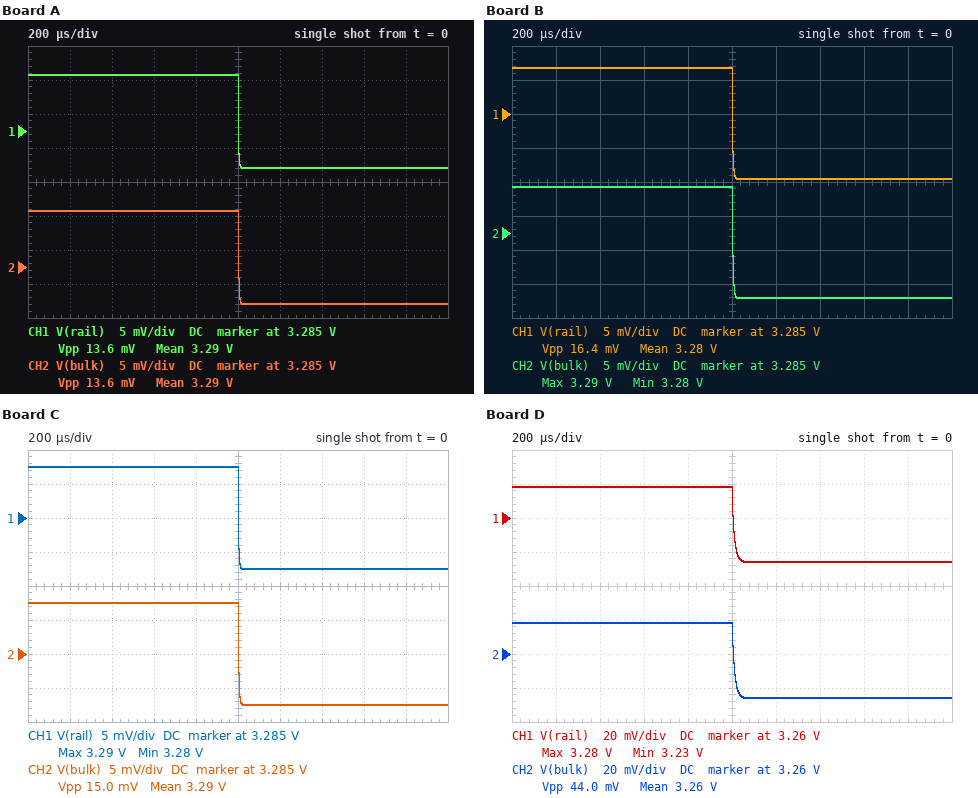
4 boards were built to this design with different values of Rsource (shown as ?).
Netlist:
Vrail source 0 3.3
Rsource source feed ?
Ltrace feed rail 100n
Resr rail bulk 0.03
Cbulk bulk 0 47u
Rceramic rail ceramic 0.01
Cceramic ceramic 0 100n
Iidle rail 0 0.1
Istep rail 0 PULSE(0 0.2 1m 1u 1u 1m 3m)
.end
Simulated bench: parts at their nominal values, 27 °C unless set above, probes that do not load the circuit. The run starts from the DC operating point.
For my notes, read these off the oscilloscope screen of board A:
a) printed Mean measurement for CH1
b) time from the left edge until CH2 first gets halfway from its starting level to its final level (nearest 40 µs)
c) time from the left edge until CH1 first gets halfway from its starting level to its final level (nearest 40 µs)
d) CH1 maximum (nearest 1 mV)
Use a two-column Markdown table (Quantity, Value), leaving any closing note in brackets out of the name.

| Quantity | Value |
|---|---|
| printed Mean measurement for CH1 | 3.29 V |
| time from the left edge until CH2 first gets halfway from its starting level to its final level | 1.00 ms |
| time from the left edge until CH1 first gets halfway from its starting level to its final level | 1.00 ms |
| CH1 maximum | 3.293 V |
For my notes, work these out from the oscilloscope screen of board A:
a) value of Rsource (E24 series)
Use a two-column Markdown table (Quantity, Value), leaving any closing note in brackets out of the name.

| Quantity | Value |
|---|---|
| value of Rsource | 0.068 Ω |
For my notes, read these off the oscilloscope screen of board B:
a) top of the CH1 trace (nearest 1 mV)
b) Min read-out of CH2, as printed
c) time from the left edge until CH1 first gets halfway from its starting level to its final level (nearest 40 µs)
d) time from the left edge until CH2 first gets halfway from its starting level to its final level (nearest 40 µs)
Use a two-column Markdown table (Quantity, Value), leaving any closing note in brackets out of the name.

| Quantity | Value |
|---|---|
| top of the CH1 trace | 3.292 V |
| Min read-out of CH2, as printed | 3.28 V |
| time from the left edge until CH1 first gets halfway from its starting level to its final level | 1.00 ms |
| time from the left edge until CH2 first gets halfway from its starting level to its final level | 1.00 ms |
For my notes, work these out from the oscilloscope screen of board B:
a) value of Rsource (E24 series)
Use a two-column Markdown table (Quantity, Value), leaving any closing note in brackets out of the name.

| Quantity | Value |
|---|---|
| value of Rsource | 0.082 Ω |
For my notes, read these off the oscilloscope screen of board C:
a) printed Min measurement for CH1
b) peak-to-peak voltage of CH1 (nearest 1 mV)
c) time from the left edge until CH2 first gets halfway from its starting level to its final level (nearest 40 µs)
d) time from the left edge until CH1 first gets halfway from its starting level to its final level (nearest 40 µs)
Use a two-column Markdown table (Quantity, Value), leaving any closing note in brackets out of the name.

| Quantity | Value |
|---|---|
| printed Min measurement for CH1 | 3.28 V |
| peak-to-peak voltage of CH1 | 15 mV |
| time from the left edge until CH2 first gets halfway from its starting level to its final level | 1.00 ms |
| time from the left edge until CH1 first gets halfway from its starting level to its final level | 1.00 ms |
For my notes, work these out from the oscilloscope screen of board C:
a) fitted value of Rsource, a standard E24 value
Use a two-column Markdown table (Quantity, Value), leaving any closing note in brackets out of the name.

| Quantity | Value |
|---|---|
| fitted value of Rsource, a standard E24 value | 0.075 Ω |
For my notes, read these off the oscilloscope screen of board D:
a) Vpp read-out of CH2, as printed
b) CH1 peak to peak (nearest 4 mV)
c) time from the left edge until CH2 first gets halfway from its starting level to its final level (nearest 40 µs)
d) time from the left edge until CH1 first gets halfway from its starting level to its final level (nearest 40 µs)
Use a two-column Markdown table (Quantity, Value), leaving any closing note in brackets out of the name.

| Quantity | Value |
|---|---|
| Vpp read-out of CH2, as printed | 44.0 mV |
| CH1 peak to peak | 44 mV |
| time from the left edge until CH2 first gets halfway from its starting level to its final level | 1.00 ms |
| time from the left edge until CH1 first gets halfway from its starting level to its final level | 1.00 ms |
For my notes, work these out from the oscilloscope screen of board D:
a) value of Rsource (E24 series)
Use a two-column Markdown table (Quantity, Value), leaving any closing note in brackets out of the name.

| Quantity | Value |
|---|---|
| value of Rsource | 0.22 Ω |
